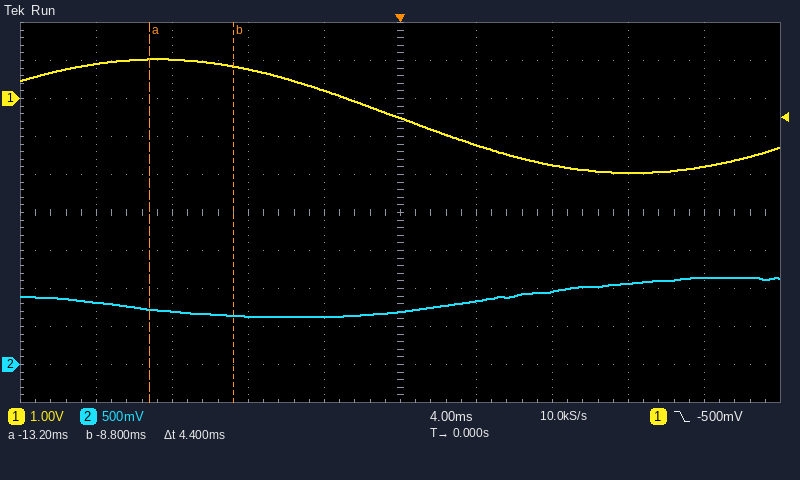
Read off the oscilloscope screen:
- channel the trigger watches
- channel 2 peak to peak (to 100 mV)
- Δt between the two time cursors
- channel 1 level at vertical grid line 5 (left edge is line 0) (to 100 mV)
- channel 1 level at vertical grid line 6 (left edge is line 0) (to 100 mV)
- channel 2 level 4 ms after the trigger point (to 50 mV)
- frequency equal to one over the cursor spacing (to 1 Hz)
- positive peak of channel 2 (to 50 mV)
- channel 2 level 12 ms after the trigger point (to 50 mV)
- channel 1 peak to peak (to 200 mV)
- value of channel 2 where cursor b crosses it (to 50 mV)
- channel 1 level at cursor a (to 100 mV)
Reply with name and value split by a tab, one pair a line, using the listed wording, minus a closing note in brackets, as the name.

channel the trigger watches	channel 1
channel 2 peak to peak	500 mV
Δt between the two time cursors	4.4 ms
channel 1 level at vertical grid line 5 (left edge is line 0)	-500 mV
channel 1 level at vertical grid line 6 (left edge is line 0)	-1.2 V
channel 2 level 4 ms after the trigger point	850 mV
frequency equal to one over the cursor spacing	227 Hz
positive peak of channel 2	1.15 V
channel 2 level 12 ms after the trigger point	1.05 V
channel 1 peak to peak	3.0 V
value of channel 2 where cursor b crosses it	650 mV
channel 1 level at cursor a	1.0 V
